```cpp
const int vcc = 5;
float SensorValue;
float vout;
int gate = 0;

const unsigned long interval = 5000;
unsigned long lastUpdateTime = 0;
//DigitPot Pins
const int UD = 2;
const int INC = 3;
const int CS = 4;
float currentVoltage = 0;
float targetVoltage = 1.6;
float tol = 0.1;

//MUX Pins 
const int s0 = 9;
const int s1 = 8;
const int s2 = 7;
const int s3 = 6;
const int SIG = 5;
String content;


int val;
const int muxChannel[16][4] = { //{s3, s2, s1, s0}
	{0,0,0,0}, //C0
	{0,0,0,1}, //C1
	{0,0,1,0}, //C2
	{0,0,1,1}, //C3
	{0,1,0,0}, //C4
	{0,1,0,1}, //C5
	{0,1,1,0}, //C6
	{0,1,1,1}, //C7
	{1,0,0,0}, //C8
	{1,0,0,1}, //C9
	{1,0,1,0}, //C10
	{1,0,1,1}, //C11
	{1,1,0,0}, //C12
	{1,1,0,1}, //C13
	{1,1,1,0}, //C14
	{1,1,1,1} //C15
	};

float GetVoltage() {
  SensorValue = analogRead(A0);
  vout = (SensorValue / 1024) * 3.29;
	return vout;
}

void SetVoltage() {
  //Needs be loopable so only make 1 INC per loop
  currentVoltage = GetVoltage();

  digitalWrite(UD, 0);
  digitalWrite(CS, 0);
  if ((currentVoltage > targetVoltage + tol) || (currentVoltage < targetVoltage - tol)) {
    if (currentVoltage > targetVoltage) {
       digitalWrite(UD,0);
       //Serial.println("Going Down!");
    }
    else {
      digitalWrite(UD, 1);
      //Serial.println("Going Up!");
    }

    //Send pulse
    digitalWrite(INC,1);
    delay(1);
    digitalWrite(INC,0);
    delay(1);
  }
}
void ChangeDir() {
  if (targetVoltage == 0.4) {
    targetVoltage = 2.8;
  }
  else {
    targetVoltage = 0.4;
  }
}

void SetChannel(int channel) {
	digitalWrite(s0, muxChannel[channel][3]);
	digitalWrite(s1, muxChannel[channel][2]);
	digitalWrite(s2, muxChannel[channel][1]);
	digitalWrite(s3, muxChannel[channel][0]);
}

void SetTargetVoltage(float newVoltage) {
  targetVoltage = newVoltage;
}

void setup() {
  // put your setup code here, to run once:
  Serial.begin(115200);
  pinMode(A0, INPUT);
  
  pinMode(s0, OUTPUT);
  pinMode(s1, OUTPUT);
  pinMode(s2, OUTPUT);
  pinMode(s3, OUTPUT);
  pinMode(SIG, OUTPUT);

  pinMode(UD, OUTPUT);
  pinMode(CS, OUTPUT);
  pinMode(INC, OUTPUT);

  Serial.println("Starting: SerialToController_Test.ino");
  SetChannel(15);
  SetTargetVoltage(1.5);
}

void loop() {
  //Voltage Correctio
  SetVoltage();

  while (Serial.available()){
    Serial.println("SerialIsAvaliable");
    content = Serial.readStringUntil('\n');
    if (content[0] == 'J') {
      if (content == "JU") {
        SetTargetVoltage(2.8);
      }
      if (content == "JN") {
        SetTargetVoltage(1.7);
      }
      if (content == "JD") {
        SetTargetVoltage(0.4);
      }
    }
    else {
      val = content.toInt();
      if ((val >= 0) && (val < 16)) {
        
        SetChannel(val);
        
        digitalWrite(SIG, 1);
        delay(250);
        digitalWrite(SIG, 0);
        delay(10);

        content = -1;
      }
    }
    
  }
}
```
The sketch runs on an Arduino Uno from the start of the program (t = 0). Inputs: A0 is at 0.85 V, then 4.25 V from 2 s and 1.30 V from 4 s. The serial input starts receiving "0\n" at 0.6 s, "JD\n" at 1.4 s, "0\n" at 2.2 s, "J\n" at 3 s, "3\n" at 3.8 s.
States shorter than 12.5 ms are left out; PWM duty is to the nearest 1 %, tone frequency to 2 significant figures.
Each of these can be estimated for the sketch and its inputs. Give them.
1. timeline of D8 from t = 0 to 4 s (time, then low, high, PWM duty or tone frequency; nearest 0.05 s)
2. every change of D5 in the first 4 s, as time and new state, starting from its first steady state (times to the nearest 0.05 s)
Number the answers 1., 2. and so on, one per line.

1. 0 s high; 0.6 s low; 3.8 s high
2. 0 s low; 0.6 s high; 0.85 s low; 2.2 s high; 2.45 s low; 3.8 s high
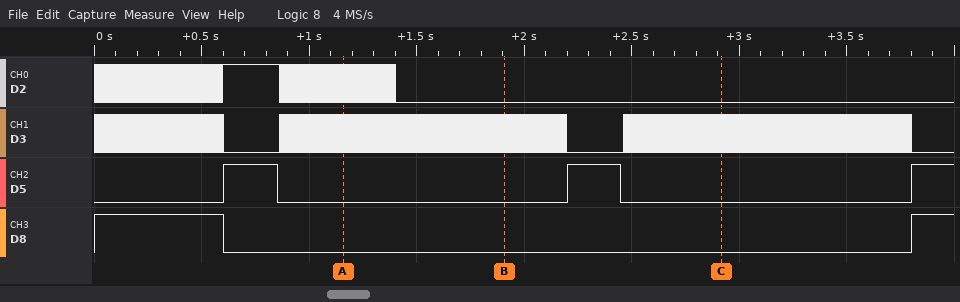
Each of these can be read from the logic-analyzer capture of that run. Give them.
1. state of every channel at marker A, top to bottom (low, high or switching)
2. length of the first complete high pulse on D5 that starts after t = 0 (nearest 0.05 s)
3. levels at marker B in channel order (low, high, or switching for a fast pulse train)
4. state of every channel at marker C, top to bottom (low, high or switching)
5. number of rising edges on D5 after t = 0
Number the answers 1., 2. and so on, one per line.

1. D2 switching, D3 switching, D5 low, D8 low
2. 0.25 s
3. D2 low, D3 switching, D5 low, D8 low
4. D2 low, D3 switching, D5 low, D8 low
5. 3
